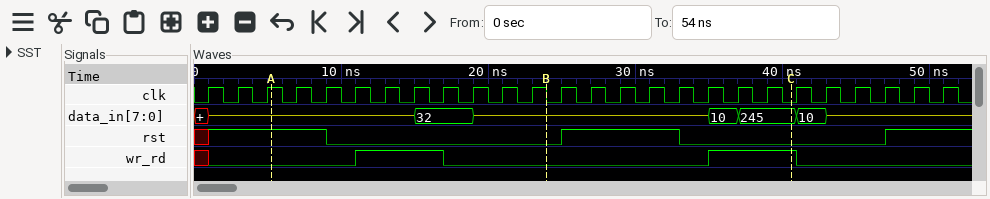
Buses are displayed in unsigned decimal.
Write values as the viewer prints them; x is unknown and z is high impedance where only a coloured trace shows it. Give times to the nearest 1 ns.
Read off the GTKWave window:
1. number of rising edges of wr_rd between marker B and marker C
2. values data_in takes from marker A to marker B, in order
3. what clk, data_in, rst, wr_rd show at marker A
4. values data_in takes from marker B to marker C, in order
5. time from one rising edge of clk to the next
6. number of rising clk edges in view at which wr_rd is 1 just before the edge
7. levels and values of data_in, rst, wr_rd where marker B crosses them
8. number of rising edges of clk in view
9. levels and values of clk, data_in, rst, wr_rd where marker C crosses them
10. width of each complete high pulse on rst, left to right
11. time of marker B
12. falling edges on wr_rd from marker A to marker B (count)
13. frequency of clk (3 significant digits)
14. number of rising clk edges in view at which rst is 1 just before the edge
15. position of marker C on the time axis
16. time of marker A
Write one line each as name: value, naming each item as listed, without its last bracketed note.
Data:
number of rising edges of wr_rd between marker B and marker C: 1
values data_in takes from marker A to marker B, in order: z, 32, z
what clk, data_in, rst, wr_rd show at marker A: clk=1, data_in=z, rst=1, wr_rd=0
values data_in takes from marker B to marker C, in order: z, 10, 245
time from one rising edge of clk to the next: 2 ns
number of rising clk edges in view at which wr_rd is 1 just before the edge: 6
levels and values of data_in, rst, wr_rd where marker B crosses them: data_in=z, rst=0, wr_rd=0
number of rising edges of clk in view: 26
levels and values of clk, data_in, rst, wr_rd where marker C crosses them: clk=0, data_in=245, rst=0, wr_rd=1
width of each complete high pulse on rst, left to right: 8 ns
time of marker B: 24 ns
falling edges on wr_rd from marker A to marker B: 1
frequency of clk: 500 MHz
number of rising clk edges in view at which rst is 1 just before the edge: 10
position of marker C on the time axis: 41 ns
time of marker A: 5 ns
